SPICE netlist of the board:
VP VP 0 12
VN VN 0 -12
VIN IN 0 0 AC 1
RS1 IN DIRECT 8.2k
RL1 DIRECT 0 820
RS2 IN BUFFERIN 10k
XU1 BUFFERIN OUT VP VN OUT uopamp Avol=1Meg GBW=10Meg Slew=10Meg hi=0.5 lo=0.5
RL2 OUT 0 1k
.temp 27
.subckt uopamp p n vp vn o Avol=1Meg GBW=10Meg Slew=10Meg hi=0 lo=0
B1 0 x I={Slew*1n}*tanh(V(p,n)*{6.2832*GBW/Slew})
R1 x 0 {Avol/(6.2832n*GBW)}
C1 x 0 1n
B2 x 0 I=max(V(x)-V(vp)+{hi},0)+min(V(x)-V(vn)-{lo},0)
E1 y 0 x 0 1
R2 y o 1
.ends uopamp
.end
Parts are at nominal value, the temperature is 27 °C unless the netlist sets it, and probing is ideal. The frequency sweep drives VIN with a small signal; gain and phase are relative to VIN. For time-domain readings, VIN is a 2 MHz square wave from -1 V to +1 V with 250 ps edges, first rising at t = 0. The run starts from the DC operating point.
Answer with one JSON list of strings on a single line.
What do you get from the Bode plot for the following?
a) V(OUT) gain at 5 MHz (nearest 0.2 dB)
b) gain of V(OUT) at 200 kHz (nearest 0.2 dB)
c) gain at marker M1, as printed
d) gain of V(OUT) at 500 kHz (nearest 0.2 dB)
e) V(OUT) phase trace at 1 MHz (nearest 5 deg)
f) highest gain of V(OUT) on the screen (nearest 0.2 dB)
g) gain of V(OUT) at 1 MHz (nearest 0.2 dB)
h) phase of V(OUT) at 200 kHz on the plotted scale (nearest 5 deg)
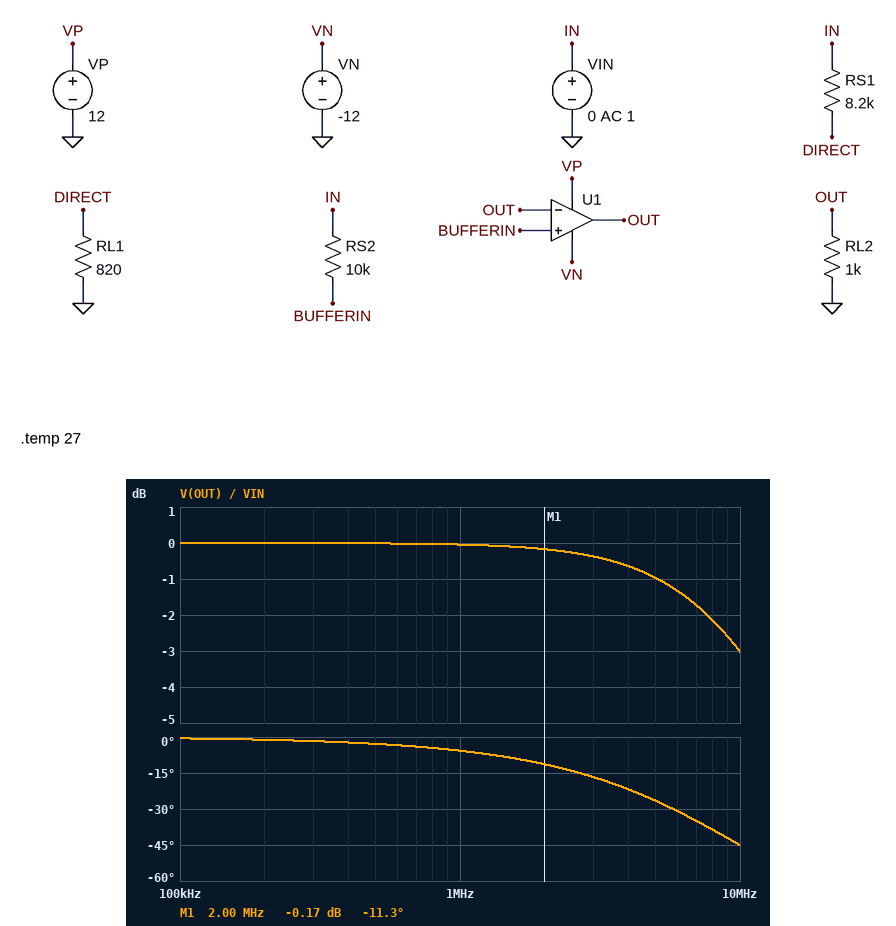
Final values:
["-1.0 dB", "0 dB", "-0.17 dB", "0 dB", "-5 deg", "0 dB", "0 dB", "0 deg"]
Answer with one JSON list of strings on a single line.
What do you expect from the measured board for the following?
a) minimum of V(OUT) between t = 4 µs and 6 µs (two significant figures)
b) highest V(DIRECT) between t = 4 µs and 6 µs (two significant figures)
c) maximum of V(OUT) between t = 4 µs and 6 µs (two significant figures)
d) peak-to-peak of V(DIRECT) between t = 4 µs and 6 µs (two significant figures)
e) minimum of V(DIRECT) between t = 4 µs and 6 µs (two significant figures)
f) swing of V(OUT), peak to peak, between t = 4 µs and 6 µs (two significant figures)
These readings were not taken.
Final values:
["-1.0 V", "91 mV", "1.0 V", "180 mV", "-91 mV", "2.0 V"]
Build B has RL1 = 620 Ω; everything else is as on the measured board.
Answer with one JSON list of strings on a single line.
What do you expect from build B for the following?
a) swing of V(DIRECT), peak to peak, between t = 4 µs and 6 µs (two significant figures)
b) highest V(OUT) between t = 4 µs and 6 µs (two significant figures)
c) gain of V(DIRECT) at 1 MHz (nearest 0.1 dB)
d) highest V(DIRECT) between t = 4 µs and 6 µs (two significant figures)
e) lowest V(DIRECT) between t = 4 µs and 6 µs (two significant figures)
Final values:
["140 mV", "1.0 V", "-23.1 dB", "70 mV", "-70 mV"]
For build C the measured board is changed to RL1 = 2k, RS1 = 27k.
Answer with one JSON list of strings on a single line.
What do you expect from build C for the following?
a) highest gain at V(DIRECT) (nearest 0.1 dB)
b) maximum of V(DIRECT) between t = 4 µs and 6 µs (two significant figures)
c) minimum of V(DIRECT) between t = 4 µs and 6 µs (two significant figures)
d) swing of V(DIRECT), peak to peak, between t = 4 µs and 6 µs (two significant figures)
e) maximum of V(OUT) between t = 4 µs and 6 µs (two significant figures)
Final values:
["-23.2 dB", "69 mV", "-69 mV", "140 mV", "1.0 V"]
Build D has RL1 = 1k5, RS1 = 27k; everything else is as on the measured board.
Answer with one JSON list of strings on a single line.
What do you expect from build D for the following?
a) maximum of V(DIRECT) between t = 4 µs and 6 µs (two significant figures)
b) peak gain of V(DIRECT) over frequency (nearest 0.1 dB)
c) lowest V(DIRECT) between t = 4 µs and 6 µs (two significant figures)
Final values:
["53 mV", "-25.6 dB", "-53 mV"]
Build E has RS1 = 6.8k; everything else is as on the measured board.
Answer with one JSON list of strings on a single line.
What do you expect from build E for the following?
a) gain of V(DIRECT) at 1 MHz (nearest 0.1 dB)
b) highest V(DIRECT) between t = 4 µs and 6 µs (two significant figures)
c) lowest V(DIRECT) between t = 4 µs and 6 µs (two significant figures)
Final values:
["-19.4 dB", "110 mV", "-110 mV"]
